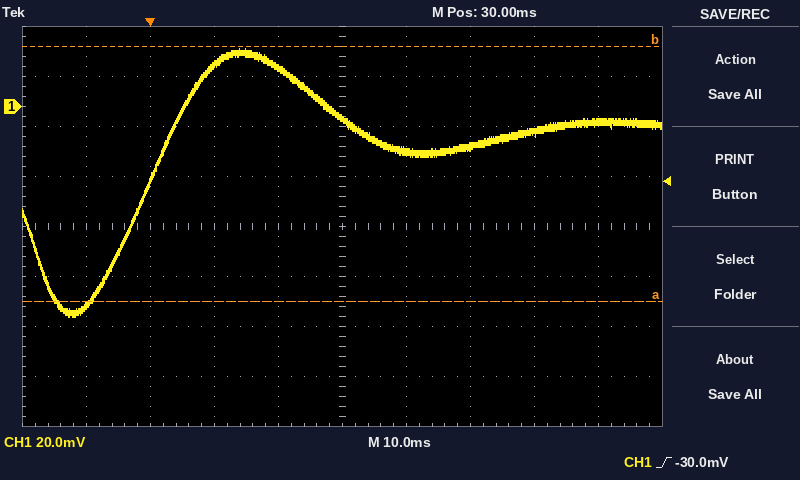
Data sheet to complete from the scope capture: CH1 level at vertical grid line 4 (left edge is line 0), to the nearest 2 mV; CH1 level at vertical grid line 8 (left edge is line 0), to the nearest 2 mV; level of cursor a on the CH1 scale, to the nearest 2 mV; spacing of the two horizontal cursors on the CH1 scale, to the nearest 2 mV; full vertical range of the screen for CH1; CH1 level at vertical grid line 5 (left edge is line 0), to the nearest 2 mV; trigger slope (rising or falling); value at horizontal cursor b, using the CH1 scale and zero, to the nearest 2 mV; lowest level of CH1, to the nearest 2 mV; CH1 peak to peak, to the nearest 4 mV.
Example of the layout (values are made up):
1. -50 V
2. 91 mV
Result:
1. 16 mV
2. -10 mV
3. -78 mV
4. 102 mV
5. 160 mV
6. -4 mV
7. rising
8. 24 mV
9. -84 mV
10. 108 mV
